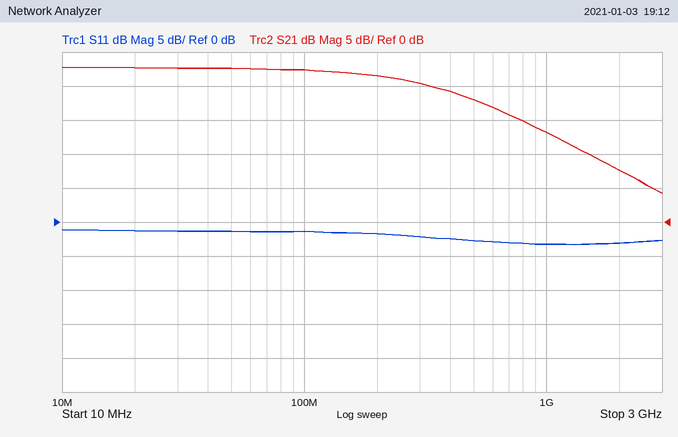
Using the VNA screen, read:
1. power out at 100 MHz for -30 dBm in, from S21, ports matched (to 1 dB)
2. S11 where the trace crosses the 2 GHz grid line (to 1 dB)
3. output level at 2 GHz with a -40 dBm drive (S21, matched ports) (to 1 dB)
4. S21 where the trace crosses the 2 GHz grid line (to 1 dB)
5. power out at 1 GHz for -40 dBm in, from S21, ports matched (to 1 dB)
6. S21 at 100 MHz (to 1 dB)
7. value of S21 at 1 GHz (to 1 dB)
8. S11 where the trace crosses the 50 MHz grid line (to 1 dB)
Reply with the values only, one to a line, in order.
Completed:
-8 dBm
-3 dB
-32 dBm
8 dB
-27 dBm
22 dB
13 dB
-1 dB
